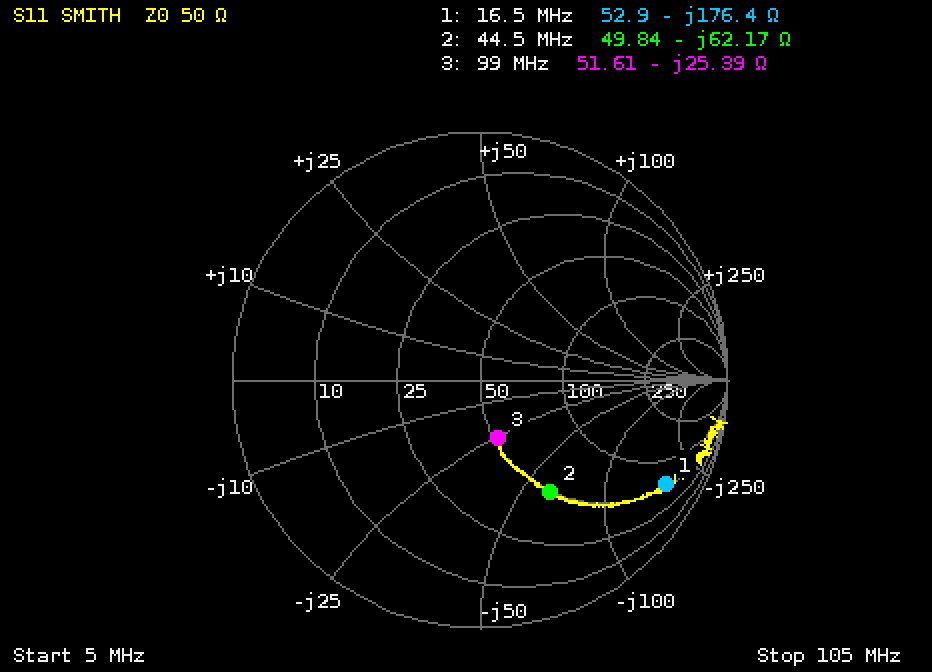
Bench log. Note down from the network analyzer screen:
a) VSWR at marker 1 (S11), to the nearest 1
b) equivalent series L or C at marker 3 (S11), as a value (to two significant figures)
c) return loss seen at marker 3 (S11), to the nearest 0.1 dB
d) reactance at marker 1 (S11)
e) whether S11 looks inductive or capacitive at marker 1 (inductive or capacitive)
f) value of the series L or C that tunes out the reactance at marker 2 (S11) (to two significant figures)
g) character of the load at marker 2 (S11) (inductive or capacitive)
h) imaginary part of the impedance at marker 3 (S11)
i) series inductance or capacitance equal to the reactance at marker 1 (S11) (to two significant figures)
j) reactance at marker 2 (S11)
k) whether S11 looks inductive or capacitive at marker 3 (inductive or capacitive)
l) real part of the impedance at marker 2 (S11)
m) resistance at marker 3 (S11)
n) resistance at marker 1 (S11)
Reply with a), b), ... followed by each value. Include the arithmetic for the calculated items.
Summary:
a) 14
b) C = 1/(2π × 99 MHz × 25.39 Ω) ≈ 63 pF
c) 12.3 dB
d) -176.4 Ω
e) capacitive
f) L = 62.17 Ω/(2π × 44.5 MHz) ≈ 222 nH, so 220 nH to two significant figures
g) capacitive
h) -25.39 Ω
i) C = 1/(2π × 16.5 MHz × 176.4 Ω) ≈ 55 pF
j) -62.17 Ω
k) capacitive
l) 49.84 Ω
m) 51.61 Ω
n) 52.9 Ω
